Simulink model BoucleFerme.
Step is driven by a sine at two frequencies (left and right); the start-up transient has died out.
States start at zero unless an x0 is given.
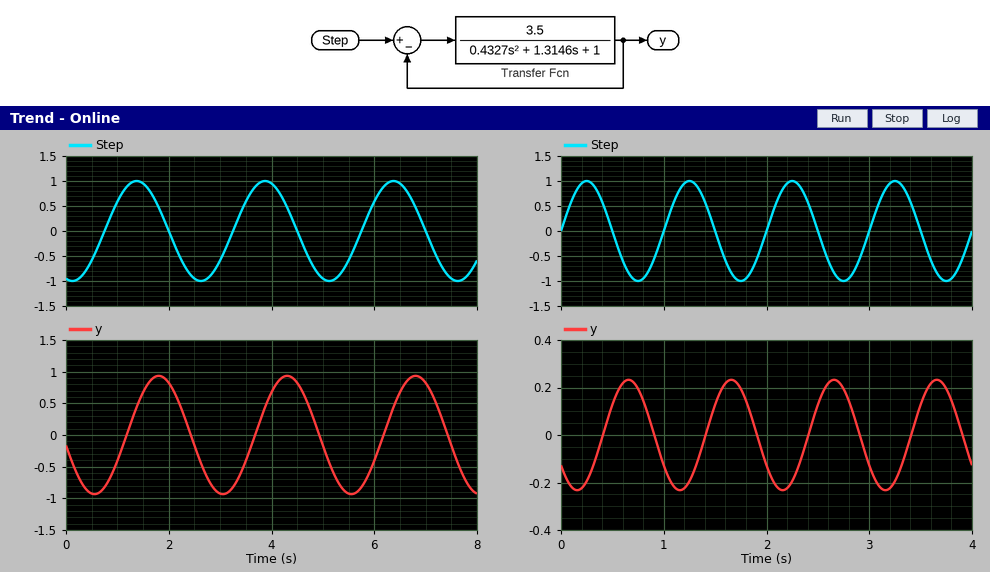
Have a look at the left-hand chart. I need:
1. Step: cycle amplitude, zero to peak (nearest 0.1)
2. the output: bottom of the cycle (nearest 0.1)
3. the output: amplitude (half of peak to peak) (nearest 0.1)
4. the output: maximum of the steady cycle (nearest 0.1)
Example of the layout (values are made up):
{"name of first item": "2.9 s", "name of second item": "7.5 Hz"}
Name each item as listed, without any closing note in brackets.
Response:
{"Step: cycle amplitude, zero to peak": "1.0", "the output: bottom of the cycle": "-0.9", "the output: amplitude (half of peak to peak)": "0.9", "the output: maximum of the steady cycle": "0.9"}
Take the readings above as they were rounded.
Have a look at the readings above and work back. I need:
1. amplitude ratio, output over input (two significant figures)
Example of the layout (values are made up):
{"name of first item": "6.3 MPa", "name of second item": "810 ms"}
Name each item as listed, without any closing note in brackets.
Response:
{"amplitude ratio, output over input": "0.90"}
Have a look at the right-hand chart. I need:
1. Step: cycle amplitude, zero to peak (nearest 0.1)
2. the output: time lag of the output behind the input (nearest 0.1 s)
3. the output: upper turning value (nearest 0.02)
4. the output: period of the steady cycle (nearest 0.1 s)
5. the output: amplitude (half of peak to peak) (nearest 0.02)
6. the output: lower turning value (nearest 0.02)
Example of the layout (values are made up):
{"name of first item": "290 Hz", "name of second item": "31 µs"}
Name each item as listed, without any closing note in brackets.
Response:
{"Step: cycle amplitude, zero to peak": "1.0", "the output: time lag of the output behind the input": "0.4 s", "the output: upper turning value": "0.24", "the output: period of the steady cycle": "1.0 s", "the output: amplitude (half of peak to peak)": "0.24", "the output: lower turning value": "-0.24"}
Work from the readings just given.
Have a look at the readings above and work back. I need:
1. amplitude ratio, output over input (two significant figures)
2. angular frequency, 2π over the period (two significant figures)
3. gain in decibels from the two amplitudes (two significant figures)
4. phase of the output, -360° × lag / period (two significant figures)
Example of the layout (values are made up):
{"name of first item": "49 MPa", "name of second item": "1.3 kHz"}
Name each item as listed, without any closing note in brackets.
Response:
{"amplitude ratio, output over input": "0.24", "angular frequency, 2π over the period": "6.3 rad/s", "gain in decibels from the two amplitudes": "-12 dB", "phase of the output, -360° × lag / period": "-140°"}
